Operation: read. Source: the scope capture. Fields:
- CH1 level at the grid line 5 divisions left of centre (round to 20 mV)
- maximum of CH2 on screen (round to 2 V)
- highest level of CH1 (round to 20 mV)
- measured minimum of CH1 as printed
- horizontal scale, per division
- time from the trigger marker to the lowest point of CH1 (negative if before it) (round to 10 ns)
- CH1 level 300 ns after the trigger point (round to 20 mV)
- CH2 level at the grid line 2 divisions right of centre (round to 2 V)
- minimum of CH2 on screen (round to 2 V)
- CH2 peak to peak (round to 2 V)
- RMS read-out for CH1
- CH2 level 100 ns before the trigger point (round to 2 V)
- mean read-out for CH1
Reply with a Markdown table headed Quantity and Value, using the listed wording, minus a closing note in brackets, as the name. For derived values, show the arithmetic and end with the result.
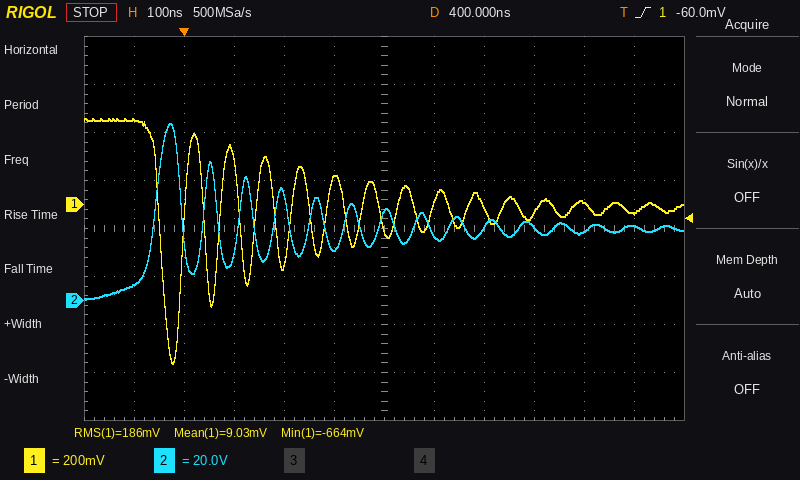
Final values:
| Quantity | Value |
|---|---|
| CH1 level at the grid line 5 divisions left of centre | 360 mV |
| maximum of CH2 on screen | 74 V |
| highest level of CH1 | 360 mV |
| measured minimum of CH1 as printed | -664 mV |
| horizontal scale, per division | 100 ns |
| time from the trigger marker to the lowest point of CH1 (negative if before it) | -20 ns |
| CH1 level 300 ns after the trigger point | 100 mV |
| CH2 level at the grid line 2 divisions right of centre | 30 V |
| minimum of CH2 on screen | 0 V |
| CH2 peak to peak | 74 V − (0 V) = 74 V |
| RMS read-out for CH1 | 186 mV |
| CH2 level 100 ns before the trigger point | 6 V |
| mean read-out for CH1 | 9.03 mV |
